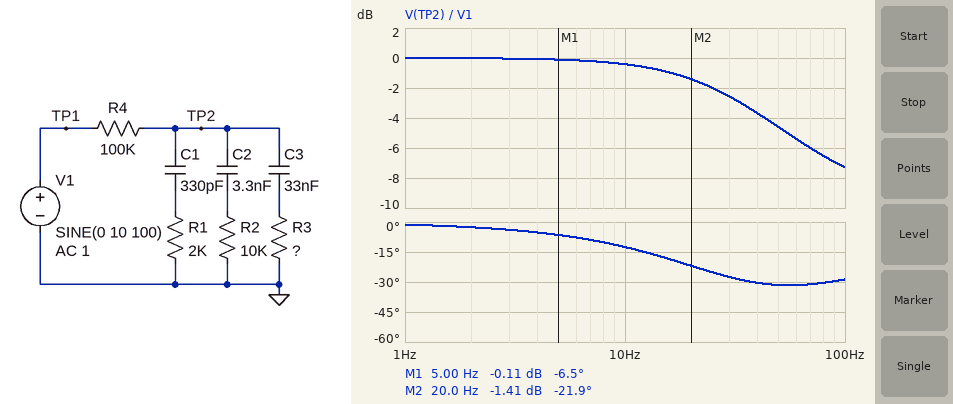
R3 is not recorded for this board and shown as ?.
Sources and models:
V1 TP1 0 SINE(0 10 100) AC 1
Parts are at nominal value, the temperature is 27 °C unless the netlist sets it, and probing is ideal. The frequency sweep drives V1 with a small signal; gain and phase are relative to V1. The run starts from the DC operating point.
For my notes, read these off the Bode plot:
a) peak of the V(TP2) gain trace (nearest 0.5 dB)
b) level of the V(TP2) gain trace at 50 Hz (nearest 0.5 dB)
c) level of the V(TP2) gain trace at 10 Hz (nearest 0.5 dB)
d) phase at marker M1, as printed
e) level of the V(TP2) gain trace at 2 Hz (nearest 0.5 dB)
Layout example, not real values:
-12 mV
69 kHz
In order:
0 dB
-4.5 dB
-0.5 dB
-6.5 deg
0 dB
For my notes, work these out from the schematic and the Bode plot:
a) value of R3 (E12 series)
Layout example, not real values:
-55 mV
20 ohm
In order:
56 kΩ
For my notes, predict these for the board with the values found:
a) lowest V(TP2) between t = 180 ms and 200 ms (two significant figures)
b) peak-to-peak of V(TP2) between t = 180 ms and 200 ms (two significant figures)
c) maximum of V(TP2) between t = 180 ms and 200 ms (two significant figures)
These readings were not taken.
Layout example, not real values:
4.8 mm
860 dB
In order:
-4.3 V
8.6 V
4.3 V
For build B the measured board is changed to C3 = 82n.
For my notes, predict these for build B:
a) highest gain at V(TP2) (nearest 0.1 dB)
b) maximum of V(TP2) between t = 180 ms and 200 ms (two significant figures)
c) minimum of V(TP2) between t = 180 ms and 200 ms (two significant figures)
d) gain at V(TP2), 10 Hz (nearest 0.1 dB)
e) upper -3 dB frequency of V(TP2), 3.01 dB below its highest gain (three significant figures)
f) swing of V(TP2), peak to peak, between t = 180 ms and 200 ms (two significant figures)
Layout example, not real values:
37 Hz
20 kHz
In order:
0 dB
3.7 V
-3.7 V
-1.9 dB
14.1 Hz
7.4 V
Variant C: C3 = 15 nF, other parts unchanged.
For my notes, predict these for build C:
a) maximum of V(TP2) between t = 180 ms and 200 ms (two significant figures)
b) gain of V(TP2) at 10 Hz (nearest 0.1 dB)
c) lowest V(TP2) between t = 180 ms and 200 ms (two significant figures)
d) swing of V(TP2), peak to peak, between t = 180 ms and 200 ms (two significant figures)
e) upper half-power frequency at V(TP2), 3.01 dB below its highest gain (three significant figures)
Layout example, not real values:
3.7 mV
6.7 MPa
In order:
5.9 V
-0.1 dB
-5.9 V
12 V
68.9 Hz
